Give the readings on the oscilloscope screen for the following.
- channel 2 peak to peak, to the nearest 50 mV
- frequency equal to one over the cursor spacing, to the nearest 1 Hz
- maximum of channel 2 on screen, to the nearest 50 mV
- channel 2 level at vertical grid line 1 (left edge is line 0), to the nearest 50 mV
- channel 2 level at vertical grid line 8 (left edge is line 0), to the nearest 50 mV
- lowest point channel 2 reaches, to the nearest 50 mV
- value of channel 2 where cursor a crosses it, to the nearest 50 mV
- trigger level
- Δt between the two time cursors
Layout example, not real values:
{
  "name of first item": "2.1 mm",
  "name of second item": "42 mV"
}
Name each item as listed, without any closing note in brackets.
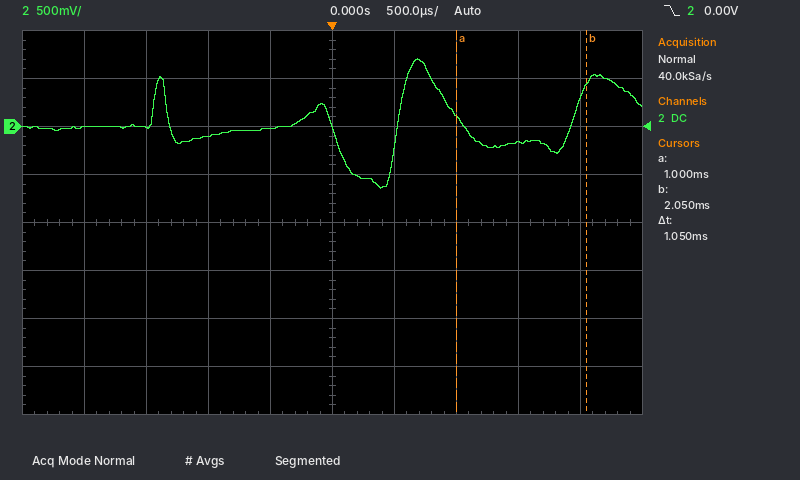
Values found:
{
  "channel 2 peak to peak, to the nearest 50 mV": "1.35 V",
  "frequency equal to one over the cursor spacing, to the nearest 1 Hz": "952 Hz",
  "maximum of channel 2 on screen, to the nearest 50 mV": "700 mV",
  "channel 2 level at vertical grid line 1 (left edge is line 0), to the nearest 50 mV": "0 mV",
  "channel 2 level at vertical grid line 8 (left edge is line 0), to the nearest 50 mV": "-150 mV",
  "lowest point channel 2 reaches, to the nearest 50 mV": "-650 mV",
  "value of channel 2 where cursor a crosses it, to the nearest 50 mV": "100 mV",
  "trigger level": "0.00 V",
  "Δt between the two time cursors": "1.05 ms"
}
